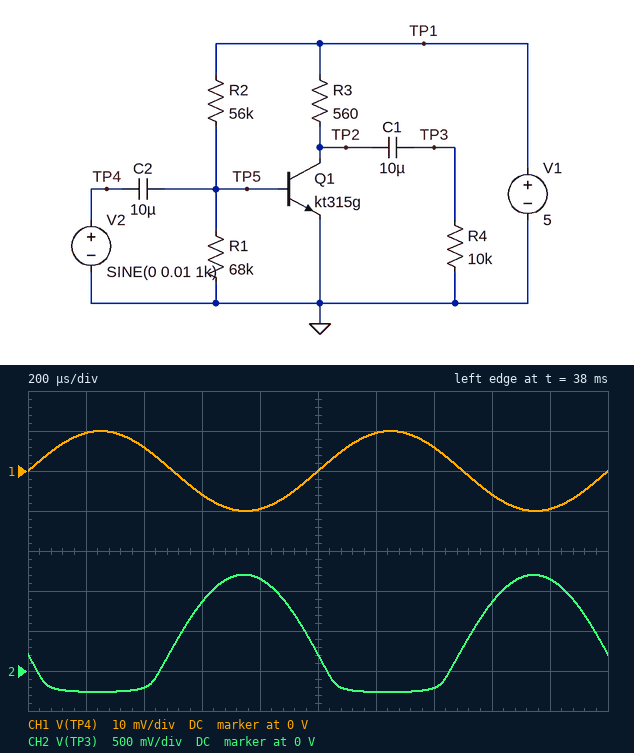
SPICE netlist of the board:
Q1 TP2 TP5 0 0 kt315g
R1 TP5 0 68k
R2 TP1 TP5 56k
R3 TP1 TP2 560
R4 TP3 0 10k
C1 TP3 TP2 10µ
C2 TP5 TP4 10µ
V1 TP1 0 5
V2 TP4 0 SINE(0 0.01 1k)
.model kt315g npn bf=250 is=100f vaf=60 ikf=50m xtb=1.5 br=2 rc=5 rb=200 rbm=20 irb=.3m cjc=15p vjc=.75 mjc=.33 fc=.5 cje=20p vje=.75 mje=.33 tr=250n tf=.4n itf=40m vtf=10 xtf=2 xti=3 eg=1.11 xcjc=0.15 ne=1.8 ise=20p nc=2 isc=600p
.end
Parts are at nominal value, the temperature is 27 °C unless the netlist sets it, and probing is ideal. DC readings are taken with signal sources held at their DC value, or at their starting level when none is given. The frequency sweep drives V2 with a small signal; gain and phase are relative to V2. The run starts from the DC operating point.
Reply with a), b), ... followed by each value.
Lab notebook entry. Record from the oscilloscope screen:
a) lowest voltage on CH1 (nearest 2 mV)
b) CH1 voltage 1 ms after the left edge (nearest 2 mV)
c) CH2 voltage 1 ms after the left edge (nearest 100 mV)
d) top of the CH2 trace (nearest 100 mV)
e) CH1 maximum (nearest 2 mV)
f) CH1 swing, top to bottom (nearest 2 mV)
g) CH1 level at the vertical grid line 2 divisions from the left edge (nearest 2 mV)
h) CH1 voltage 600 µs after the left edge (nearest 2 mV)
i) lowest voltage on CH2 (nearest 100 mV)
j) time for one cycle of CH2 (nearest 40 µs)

a) -10 mV
b) 0 V
c) 200 mV
d) 1.2 V
e) 10 mV
f) 20 mV
g) 6 mV
h) -6 mV
i) -300 mV
j) 1.00 ms
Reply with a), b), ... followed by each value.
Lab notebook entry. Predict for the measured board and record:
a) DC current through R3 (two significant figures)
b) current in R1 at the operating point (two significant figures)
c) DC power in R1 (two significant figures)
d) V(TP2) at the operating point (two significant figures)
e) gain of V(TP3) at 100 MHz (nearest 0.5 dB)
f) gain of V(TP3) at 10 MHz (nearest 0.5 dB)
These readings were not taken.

a) 8.4 mA
b) 9.8 µA
c) 6.5 µW
d) 280 mV
e) 0 dB
f) 17.5 dB
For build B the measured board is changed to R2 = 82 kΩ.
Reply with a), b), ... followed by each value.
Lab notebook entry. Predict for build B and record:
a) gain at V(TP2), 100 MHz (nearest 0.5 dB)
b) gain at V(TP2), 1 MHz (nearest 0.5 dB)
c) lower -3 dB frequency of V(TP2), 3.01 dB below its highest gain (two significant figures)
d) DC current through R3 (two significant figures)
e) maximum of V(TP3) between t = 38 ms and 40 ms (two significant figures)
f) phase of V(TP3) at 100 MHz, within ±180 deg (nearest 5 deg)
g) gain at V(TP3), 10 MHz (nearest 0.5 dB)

a) 8.0 dB
b) 38.0 dB
c) 18 Hz
d) 5.5 mA
e) 780 mV
f) 35 deg
g) 29.5 dB
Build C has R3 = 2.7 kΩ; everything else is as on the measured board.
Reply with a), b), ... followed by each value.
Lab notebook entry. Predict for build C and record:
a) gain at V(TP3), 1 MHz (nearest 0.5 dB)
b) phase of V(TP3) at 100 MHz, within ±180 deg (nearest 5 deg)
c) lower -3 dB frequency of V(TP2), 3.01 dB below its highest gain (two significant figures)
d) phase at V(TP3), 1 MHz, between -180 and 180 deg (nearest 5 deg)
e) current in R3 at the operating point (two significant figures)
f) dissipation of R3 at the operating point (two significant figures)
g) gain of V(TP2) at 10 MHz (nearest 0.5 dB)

a) 1.5 dB
b) 30 deg
c) 84 Hz
d) 110 deg
e) 1.8 mA
f) 8.9 mW
g) -15.5 dB
